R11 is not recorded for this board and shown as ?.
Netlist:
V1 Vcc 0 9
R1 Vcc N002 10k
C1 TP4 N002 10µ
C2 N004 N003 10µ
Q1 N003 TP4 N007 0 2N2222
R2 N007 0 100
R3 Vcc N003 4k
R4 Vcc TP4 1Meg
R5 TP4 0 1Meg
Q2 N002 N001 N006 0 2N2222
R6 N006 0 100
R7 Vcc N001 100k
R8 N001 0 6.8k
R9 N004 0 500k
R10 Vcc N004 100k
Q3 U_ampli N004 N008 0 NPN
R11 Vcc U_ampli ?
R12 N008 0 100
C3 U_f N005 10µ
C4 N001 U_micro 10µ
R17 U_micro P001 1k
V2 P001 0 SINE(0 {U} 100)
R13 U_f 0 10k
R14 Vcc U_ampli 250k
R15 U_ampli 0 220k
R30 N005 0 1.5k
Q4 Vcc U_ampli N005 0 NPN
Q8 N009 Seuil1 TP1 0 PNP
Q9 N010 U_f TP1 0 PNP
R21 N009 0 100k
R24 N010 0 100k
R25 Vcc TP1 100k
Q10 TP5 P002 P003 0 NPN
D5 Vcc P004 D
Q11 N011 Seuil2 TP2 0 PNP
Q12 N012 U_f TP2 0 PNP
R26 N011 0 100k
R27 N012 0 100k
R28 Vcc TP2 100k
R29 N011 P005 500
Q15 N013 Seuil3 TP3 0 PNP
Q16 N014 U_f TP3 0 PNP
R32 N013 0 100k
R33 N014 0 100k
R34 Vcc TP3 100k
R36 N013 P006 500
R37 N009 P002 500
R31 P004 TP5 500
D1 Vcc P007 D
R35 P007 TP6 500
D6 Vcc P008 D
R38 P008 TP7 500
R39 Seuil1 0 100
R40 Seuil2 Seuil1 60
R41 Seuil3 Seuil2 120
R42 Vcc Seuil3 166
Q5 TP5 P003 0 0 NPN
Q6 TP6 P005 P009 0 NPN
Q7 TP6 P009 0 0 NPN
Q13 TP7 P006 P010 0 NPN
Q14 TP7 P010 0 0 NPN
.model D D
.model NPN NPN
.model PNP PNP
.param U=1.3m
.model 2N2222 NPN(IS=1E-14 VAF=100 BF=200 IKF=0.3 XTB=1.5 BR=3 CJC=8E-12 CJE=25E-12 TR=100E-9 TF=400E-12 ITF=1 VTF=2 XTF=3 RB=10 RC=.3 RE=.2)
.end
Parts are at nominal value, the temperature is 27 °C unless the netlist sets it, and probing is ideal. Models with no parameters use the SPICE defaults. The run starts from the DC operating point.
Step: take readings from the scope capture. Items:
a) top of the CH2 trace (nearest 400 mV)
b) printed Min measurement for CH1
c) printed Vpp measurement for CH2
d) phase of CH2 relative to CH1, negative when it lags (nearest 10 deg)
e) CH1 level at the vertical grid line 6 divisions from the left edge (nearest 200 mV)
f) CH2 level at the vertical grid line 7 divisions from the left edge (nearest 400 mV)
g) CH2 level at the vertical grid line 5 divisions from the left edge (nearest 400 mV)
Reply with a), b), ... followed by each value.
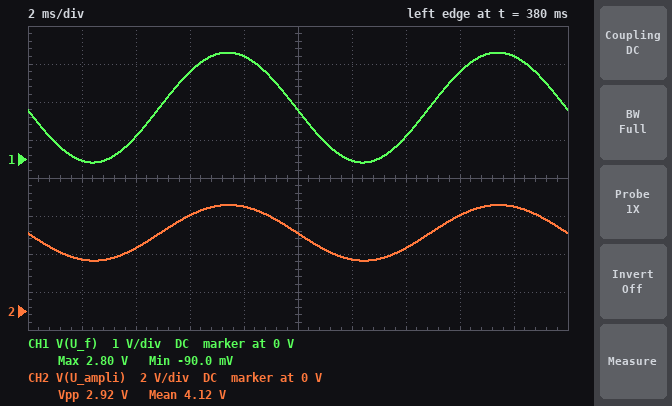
a) 5.6 V
b) -90.0 mV
c) 2.92 V
d) 0 deg
e) 0 V
f) 3.2 V
g) 4.0 V
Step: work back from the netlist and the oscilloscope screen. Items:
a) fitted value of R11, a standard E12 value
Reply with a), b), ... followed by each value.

a) 680 Ω
